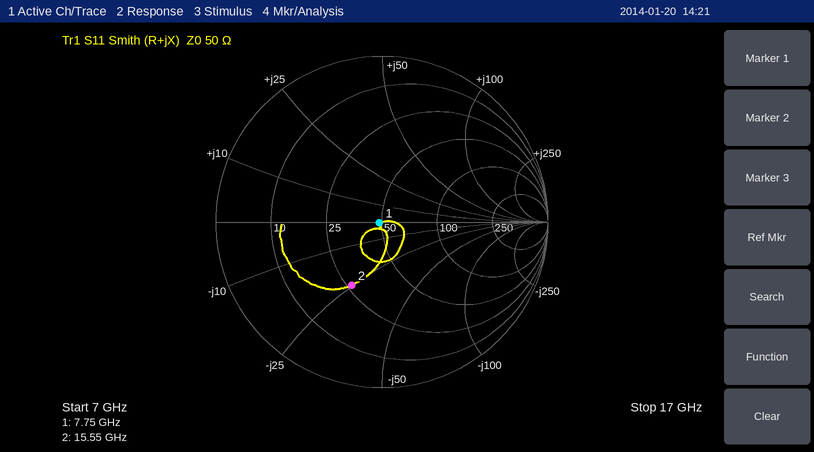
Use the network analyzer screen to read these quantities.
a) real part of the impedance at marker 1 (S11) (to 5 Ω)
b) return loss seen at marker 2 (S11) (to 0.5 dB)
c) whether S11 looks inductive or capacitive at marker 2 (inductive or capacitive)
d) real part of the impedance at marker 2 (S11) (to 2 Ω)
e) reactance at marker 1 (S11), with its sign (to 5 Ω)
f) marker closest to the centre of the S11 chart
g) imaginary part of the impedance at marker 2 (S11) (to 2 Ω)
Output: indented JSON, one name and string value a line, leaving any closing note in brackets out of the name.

{
  "real part of the impedance at marker 1 (S11)": "50 Ω",
  "return loss seen at marker 2 (S11)": "7.5 dB",
  "whether S11 looks inductive or capacitive at marker 2": "capacitive",
  "real part of the impedance at marker 2 (S11)": "26 Ω",
  "reactance at marker 1 (S11), with its sign": "0 Ω",
  "marker closest to the centre of the S11 chart": "marker 1",
  "imaginary part of the impedance at marker 2 (S11)": "-24 Ω"
}
